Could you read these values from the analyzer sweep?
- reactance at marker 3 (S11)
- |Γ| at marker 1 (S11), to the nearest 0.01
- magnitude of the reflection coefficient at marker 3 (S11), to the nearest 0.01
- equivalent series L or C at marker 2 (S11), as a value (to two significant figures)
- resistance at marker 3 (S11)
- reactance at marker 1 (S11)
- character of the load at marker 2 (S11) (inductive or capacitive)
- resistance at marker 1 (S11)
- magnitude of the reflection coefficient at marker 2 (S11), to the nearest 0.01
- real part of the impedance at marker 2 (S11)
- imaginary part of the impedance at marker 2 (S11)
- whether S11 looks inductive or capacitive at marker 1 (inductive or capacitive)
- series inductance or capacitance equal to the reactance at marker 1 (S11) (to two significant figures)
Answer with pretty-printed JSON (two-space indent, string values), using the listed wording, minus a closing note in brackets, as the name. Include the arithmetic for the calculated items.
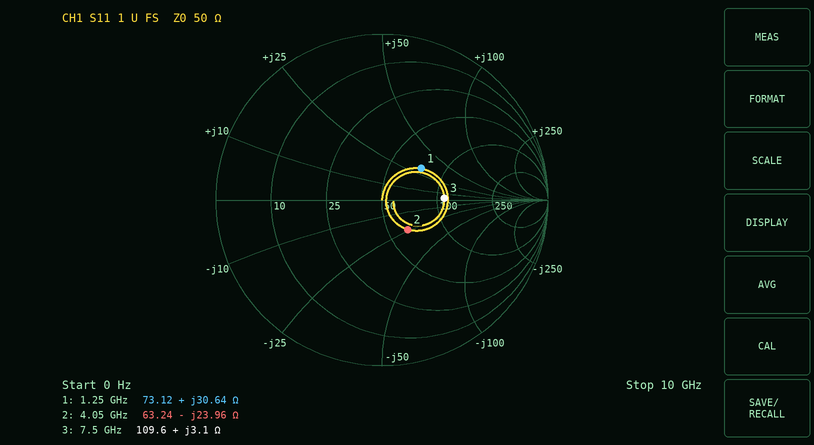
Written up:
{
  "reactance at marker 3": "+3.1 Ω",
  "|Γ| at marker 1 (S11), to the nearest 0.01": "0.30",
  "magnitude of the reflection coefficient at marker 3 (S11), to the nearest 0.01": "0.37",
  "equivalent series L or C at marker 2 (S11), as a value": "C = 1/(2π × 4.05 GHz × 23.96 Ω) ≈ 1.6 pF",
  "resistance at marker 3": "109.6 Ω",
  "reactance at marker 1": "+30.64 Ω",
  "character of the load at marker 2 (S11)": "capacitive",
  "resistance at marker 1": "73.12 Ω",
  "magnitude of the reflection coefficient at marker 2 (S11), to the nearest 0.01": "0.24",
  "real part of the impedance at marker 2": "63.24 Ω",
  "imaginary part of the impedance at marker 2": "-23.96 Ω",
  "whether S11 looks inductive or capacitive at marker 1": "inductive",
  "series inductance or capacitance equal to the reactance at marker 1 (S11)": "L = 30.64 Ω/(2π × 1.25 GHz) ≈ 3.9 nH"
}
